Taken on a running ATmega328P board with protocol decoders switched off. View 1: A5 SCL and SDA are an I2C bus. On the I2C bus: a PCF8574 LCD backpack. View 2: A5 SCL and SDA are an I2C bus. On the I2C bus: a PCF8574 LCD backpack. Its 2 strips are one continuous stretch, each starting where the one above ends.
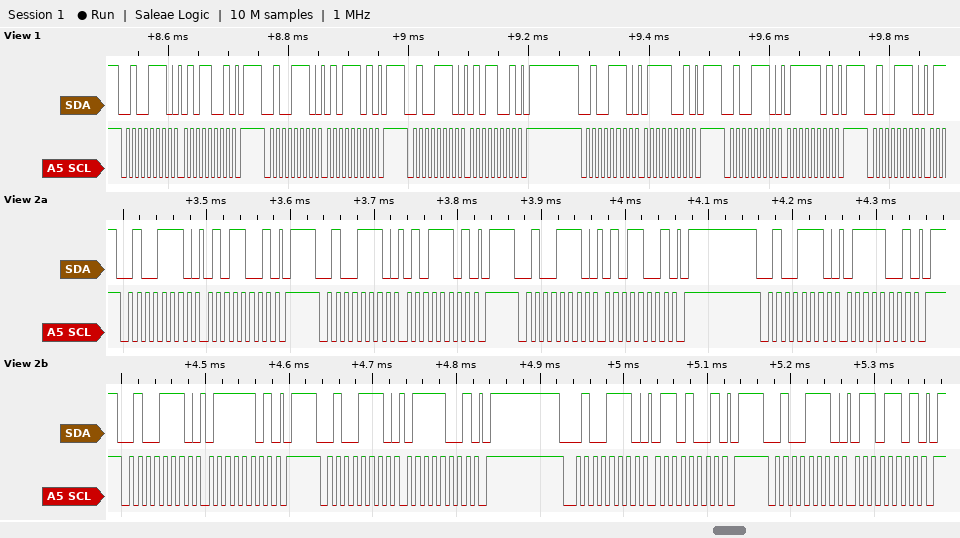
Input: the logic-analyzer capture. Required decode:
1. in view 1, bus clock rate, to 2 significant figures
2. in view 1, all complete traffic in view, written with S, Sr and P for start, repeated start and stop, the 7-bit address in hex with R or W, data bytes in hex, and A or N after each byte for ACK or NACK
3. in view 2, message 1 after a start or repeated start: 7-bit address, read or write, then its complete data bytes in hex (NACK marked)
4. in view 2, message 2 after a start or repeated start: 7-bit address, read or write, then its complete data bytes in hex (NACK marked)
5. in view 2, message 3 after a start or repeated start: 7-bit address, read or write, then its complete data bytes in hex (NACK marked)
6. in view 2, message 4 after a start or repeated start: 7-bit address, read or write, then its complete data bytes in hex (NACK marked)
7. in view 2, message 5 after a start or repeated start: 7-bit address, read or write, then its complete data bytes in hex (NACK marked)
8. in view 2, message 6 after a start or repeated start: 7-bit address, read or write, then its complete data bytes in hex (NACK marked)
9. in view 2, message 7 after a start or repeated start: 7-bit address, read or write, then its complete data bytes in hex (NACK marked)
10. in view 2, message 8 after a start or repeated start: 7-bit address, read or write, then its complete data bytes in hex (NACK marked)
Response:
100 kHz
S 27W A 59 A P S 27W A 5D A P S 27W A 59 A P S 27W A 79 A P S 27W A 7D A P S 27W A
0x27 write: 59
0x27 write: 5D
0x27 write: 59
0x27 write: 79
0x27 write: 7D
0x27 write: 79
0x27 write: 69
0x27 write: 6D
